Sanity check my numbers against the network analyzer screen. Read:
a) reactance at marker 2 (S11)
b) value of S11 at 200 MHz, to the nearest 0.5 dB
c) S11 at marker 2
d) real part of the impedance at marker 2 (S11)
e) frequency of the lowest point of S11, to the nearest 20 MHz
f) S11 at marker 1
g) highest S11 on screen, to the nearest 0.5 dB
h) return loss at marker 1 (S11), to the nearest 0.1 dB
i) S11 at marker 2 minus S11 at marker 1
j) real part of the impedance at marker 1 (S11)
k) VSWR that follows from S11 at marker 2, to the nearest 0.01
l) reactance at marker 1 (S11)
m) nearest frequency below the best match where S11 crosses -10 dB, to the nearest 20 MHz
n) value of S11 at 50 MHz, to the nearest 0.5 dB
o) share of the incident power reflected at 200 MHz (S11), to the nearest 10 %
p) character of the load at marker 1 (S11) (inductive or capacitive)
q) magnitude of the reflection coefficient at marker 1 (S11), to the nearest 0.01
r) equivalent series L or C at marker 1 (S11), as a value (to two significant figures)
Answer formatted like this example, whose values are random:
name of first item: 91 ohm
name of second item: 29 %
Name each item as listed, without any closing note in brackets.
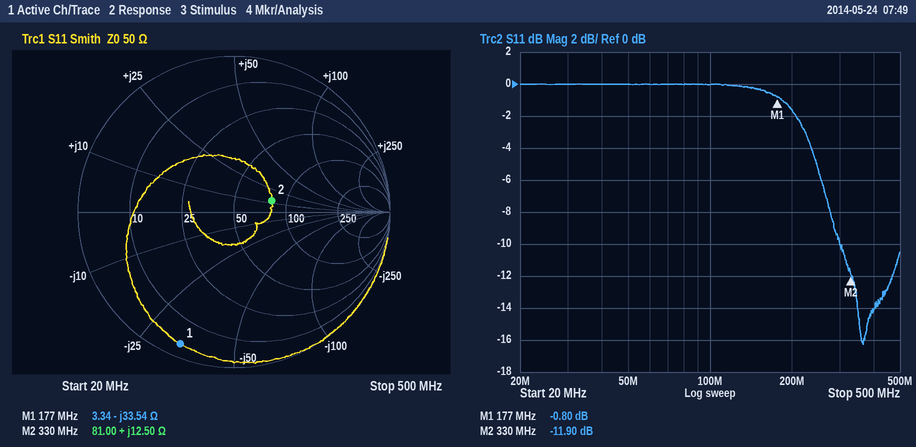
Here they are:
reactance at marker 2: +12.50 Ω
value of S11 at 200 MHz, to the nearest 0.5 dB: -1.5 dB
S11 at marker 2: -11.90 dB
real part of the impedance at marker 2: 81.00 Ω
frequency of the lowest point of S11, to the nearest 20 MHz: 360 MHz
S11 at marker 1: -0.80 dB
highest S11 on screen, to the nearest 0.5 dB: 0.0 dB
return loss at marker 1 (S11), to the nearest 0.1 dB: 0.8 dB
S11 at marker 2 minus S11 at marker 1: -11.10 dB
real part of the impedance at marker 1: 3.34 Ω
VSWR that follows from S11 at marker 2, to the nearest 0.01: 1.68
reactance at marker 1: -33.54 Ω
nearest frequency below the best match where S11 crosses -10 dB, to the nearest 20 MHz: 300 MHz
value of S11 at 50 MHz, to the nearest 0.5 dB: 0.0 dB
share of the incident power reflected at 200 MHz (S11), to the nearest 10 %: 70 %
character of the load at marker 1 (S11): capacitive
magnitude of the reflection coefficient at marker 1 (S11), to the nearest 0.01: 0.91
equivalent series L or C at marker 1 (S11), as a value: 27 pF
